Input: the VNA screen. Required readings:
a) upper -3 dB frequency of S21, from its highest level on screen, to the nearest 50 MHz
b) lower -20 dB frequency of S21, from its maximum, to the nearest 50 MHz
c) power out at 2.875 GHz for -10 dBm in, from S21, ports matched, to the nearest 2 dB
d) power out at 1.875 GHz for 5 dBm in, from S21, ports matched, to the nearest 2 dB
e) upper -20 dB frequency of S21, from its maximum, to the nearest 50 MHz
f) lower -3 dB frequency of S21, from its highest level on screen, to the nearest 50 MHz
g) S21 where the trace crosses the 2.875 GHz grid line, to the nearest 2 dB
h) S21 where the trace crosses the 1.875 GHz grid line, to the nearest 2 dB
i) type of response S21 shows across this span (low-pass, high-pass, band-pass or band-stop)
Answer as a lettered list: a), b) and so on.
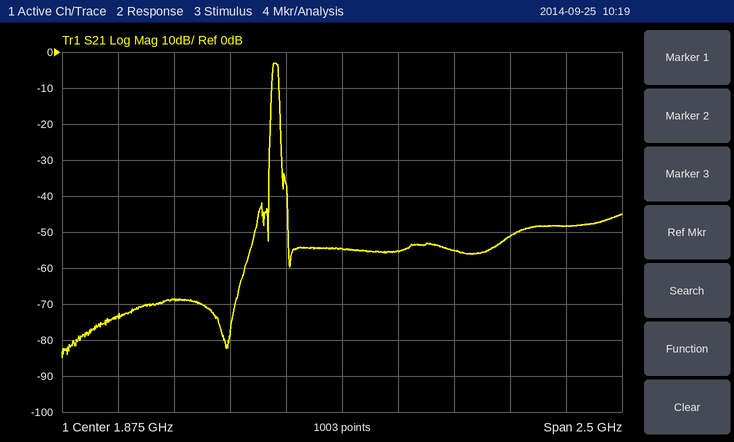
a) 1.60 GHz
b) 1.55 GHz
c) -58 dBm
d) -50 dBm
e) 1.60 GHz
f) 1.55 GHz
g) -48 dB
h) -54 dB
i) band-pass
